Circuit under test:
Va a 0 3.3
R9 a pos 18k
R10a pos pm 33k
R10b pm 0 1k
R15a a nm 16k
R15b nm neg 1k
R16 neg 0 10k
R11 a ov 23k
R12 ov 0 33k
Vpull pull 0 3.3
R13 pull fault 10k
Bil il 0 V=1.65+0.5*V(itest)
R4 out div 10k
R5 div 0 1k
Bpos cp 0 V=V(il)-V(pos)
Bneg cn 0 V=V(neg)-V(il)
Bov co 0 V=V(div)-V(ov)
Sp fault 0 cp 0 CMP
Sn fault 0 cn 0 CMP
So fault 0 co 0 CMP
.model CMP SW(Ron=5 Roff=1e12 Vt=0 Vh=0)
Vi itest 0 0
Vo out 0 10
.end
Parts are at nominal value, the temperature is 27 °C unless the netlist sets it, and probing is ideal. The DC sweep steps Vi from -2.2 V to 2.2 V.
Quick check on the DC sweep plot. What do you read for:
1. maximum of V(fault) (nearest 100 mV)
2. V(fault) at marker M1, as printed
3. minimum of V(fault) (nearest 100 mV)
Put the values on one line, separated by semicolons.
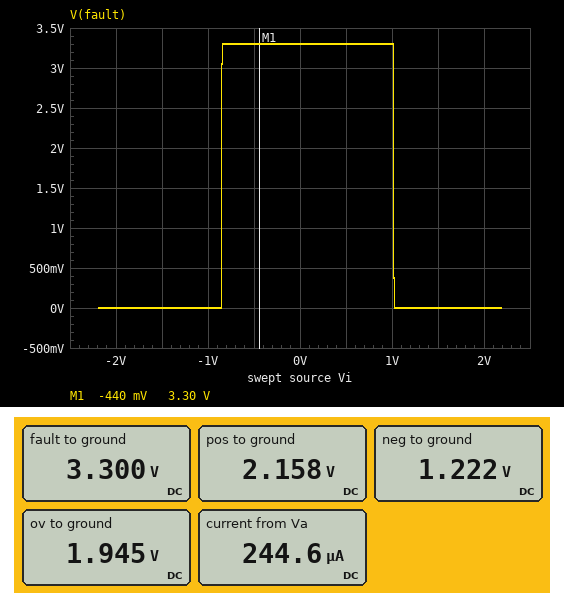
3.3 V; 3.30 V; 0 V
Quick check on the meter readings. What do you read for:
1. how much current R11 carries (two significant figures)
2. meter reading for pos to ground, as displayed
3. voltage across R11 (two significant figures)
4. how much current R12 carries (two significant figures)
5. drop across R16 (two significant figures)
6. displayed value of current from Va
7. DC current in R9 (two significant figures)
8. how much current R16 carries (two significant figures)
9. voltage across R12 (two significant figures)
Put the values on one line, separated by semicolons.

59 µA; 2.158 V; 1.4 V; 59 µA; 1.2 V; 244.6 µA; 63 µA; 120 µA; 1.9 V
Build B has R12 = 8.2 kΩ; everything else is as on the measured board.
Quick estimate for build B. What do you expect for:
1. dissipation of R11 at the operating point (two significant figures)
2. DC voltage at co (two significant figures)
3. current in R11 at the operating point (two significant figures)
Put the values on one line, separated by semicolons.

260 µW; 42 mV; 110 µA
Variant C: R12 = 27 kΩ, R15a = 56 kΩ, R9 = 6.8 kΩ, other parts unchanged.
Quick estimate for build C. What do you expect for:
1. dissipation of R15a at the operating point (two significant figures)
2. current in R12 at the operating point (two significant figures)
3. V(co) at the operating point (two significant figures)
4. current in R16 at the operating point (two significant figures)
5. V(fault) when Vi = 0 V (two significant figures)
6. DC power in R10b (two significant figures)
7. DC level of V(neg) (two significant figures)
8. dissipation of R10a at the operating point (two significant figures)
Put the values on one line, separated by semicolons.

140 µW; 66 µA; -870 mV; 49 µA; 3.3 V; 6.5 µW; 490 mV; 220 µW
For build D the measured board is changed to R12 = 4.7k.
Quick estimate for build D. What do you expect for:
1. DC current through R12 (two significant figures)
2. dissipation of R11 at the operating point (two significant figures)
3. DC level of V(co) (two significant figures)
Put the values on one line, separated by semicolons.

120 µA; 330 µW; 350 mV
